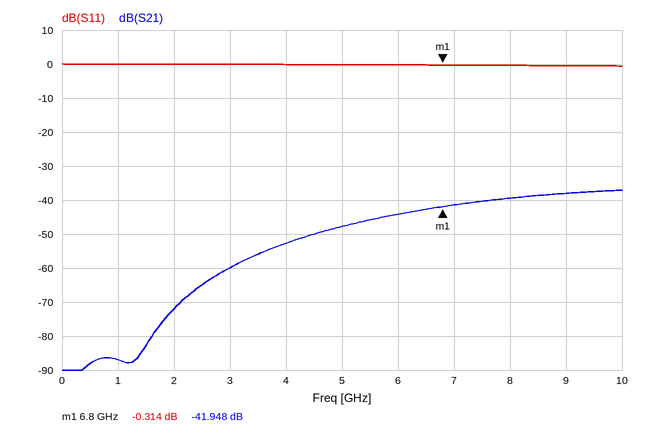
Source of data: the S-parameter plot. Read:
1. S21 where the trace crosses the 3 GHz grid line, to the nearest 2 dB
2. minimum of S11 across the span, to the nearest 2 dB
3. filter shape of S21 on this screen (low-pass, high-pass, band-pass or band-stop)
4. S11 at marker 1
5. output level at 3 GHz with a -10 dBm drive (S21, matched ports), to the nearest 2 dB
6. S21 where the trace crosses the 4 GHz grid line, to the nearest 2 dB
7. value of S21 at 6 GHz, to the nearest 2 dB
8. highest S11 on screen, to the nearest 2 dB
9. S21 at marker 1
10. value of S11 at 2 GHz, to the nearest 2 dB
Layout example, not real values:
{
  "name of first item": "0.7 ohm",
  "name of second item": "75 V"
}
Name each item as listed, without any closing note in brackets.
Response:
{
  "S21 where the trace crosses the 3 GHz grid line, to the nearest 2 dB": "-60 dB",
  "minimum of S11 across the span, to the nearest 2 dB": "0 dB",
  "filter shape of S21 on this screen": "high-pass",
  "S11 at marker 1": "-0.314 dB",
  "output level at 3 GHz with a -10 dBm drive (S21, matched ports), to the nearest 2 dB": "-70 dBm",
  "S21 where the trace crosses the 4 GHz grid line, to the nearest 2 dB": "-52 dB",
  "value of S21 at 6 GHz, to the nearest 2 dB": "-44 dB",
  "highest S11 on screen, to the nearest 2 dB": "0 dB",
  "S21 at marker 1": "-41.948 dB",
  "value of S11 at 2 GHz, to the nearest 2 dB": "0 dB"
}
